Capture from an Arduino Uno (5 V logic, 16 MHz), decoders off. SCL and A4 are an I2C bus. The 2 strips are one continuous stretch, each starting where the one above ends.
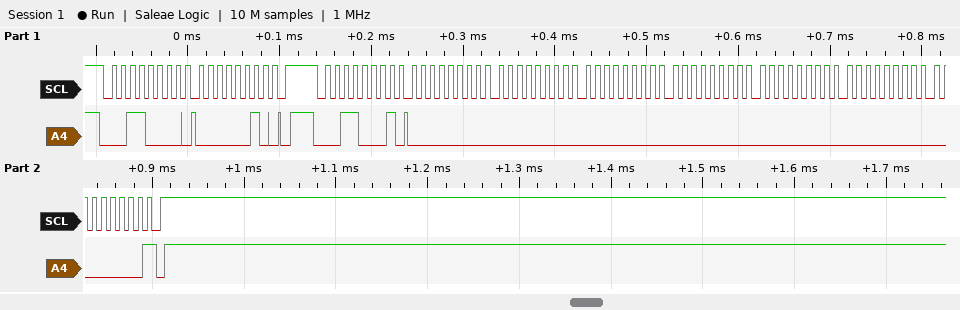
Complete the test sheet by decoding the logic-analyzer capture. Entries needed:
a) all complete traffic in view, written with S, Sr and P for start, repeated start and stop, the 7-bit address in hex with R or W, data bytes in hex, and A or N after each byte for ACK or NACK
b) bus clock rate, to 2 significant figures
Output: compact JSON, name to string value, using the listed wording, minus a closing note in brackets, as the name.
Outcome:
{"all complete traffic in view, written with S, Sr and P for start, repeated start and stop, the 7-bit address in hex with R or W, data bytes in hex, and A or N after each byte for ACK or NACK": "S 18W A 02 A P S 18R A 00 A 00 A 00 A 00 A 00 A 00 A 00 N P", "bus clock rate, to 2 significant figures": "100 kHz"}
